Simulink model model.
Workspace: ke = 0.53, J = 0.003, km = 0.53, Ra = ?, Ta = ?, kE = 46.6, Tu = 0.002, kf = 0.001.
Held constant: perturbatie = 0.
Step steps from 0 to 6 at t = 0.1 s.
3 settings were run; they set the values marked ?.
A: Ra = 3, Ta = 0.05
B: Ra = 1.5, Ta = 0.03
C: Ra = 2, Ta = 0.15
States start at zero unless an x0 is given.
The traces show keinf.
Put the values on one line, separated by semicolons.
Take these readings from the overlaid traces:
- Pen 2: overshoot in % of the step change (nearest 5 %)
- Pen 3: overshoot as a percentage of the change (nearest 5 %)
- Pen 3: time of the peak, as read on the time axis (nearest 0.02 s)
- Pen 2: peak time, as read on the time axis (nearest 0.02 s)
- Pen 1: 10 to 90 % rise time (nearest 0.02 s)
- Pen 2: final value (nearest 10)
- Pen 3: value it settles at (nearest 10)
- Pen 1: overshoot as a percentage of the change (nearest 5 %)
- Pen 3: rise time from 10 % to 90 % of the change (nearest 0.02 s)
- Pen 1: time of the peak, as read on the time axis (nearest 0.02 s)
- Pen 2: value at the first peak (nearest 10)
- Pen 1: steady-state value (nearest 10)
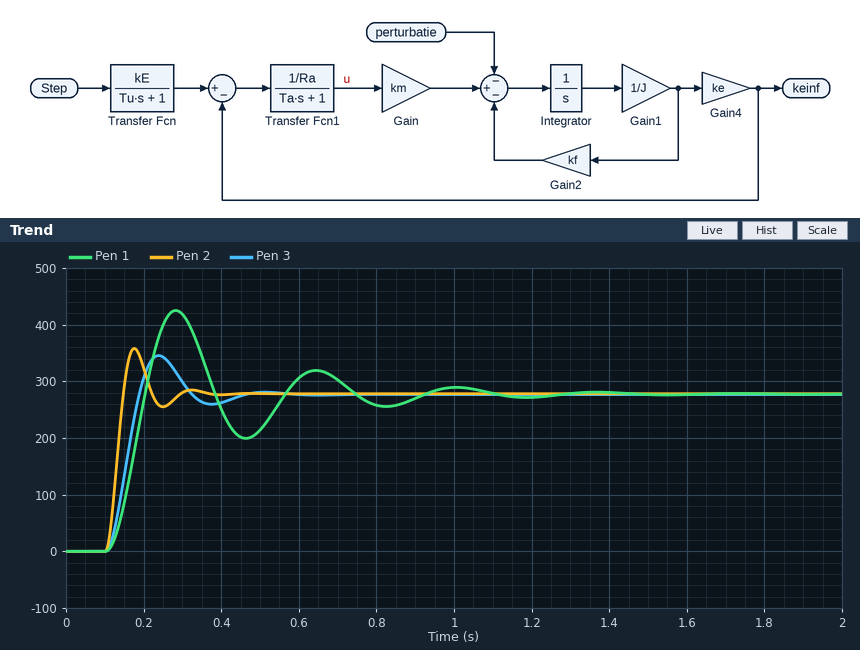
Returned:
30 %; 25 %; 0.24 s; 0.18 s; 0.06 s; 280; 280; 55 %; 0.06 s; 0.28 s; 360; 280
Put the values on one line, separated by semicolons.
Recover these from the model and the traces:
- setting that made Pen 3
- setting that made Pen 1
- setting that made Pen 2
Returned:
A; C; B
